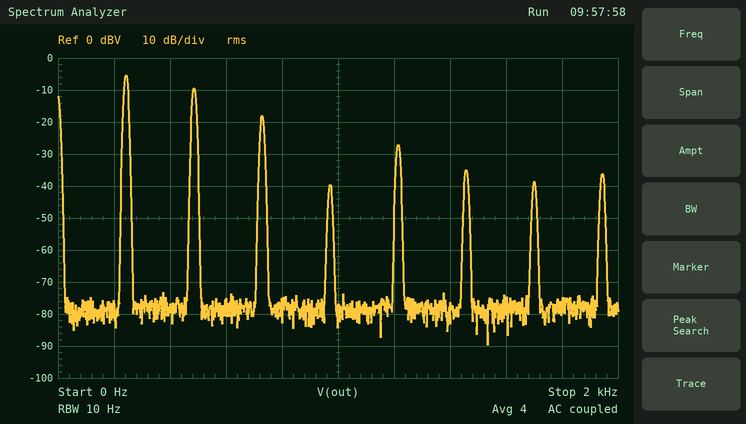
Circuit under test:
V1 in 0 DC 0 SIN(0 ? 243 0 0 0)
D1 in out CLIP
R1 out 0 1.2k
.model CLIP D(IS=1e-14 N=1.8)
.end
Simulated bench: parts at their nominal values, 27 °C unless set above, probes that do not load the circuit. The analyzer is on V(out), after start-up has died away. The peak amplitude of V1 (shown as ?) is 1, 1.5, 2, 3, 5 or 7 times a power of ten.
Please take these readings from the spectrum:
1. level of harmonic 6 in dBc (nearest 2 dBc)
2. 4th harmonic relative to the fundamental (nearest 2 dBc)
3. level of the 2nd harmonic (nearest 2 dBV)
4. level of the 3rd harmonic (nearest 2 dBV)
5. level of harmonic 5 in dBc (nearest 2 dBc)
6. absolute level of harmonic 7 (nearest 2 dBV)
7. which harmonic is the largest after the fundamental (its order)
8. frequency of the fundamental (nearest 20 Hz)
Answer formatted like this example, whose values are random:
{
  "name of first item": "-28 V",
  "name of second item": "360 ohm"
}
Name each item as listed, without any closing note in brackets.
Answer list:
{
  "level of harmonic 6 in dBc": "-30 dBc",
  "4th harmonic relative to the fundamental": "-34 dBc",
  "level of the 2nd harmonic": "-10 dBV",
  "level of the 3rd harmonic": "-18 dBV",
  "level of harmonic 5 in dBc": "-22 dBc",
  "absolute level of harmonic 7": "-38 dBV",
  "which harmonic is the largest after the fundamental": "2",
  "frequency of the fundamental": "240 Hz"
}
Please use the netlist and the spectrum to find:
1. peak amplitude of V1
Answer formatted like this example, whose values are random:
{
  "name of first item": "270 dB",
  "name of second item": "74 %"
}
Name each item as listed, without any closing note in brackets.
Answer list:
{
  "peak amplitude of V1": "3 V"
}
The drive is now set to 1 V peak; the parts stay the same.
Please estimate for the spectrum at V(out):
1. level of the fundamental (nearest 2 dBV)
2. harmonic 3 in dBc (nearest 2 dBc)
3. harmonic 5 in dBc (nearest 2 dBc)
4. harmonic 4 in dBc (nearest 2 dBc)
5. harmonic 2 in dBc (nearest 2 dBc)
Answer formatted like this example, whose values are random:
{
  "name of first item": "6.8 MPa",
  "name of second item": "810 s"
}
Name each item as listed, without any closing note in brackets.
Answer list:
{
  "level of the fundamental": "-52 dBV",
  "harmonic 3 in dBc": "-2 dBc",
  "harmonic 5 in dBc": "-6 dBc",
  "harmonic 4 in dBc": "-4 dBc",
  "harmonic 2 in dBc": "0 dBc"
}
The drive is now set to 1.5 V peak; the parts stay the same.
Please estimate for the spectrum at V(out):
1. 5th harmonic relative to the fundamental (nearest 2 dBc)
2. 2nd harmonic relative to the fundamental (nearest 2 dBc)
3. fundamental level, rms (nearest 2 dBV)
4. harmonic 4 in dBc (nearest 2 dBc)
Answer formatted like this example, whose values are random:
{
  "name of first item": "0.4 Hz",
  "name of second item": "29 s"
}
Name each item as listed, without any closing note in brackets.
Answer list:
{
  "5th harmonic relative to the fundamental": "-20 dBc",
  "2nd harmonic relative to the fundamental": "-2 dBc",
  "fundamental level, rms": "-22 dBV",
  "harmonic 4 in dBc": "-10 dBc"
}
